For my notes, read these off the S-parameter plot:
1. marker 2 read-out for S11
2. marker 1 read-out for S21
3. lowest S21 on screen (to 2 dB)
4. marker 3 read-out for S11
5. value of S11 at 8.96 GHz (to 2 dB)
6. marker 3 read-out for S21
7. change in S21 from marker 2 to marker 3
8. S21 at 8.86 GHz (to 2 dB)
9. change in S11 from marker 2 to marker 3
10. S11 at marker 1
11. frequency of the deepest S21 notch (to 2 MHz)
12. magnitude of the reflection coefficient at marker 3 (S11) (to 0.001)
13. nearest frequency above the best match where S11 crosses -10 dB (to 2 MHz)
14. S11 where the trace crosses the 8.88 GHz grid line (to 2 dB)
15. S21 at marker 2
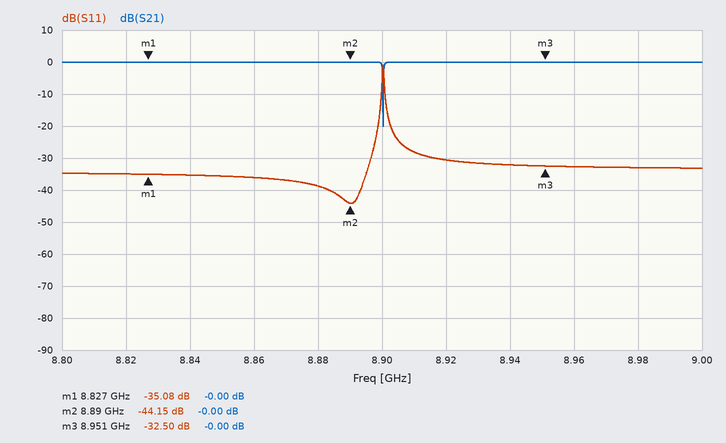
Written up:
-44.15 dB
-0.00 dB
-20 dB
-32.50 dB
-32 dB
-0.00 dB
0.00 dB
0 dB
11.65 dB
-35.08 dB
8.900 GHz
0.024
8.900 GHz
-38 dB
-0.00 dB
